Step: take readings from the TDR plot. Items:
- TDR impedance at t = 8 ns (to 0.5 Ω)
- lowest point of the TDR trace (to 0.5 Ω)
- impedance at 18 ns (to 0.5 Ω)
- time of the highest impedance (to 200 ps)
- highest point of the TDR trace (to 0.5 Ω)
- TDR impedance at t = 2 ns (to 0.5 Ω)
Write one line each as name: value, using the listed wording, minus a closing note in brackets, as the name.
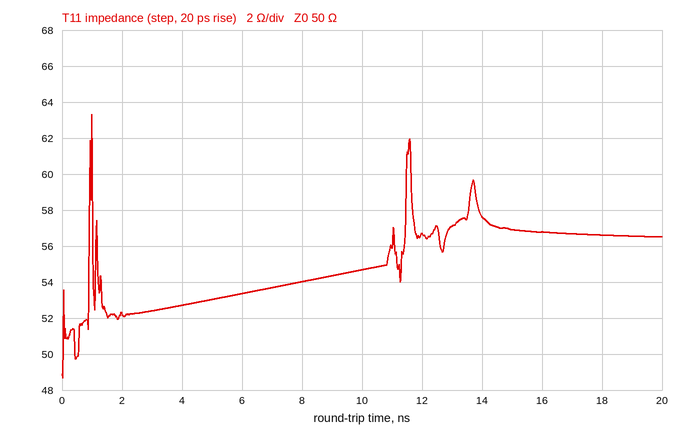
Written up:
TDR impedance at t = 8 ns: 54.0 Ω
lowest point of the TDR trace: 48.5 Ω
impedance at 18 ns: 56.5 Ω
time of the highest impedance: 1.0 ns
highest point of the TDR trace: 63.5 Ω
TDR impedance at t = 2 ns: 52.0 Ω
